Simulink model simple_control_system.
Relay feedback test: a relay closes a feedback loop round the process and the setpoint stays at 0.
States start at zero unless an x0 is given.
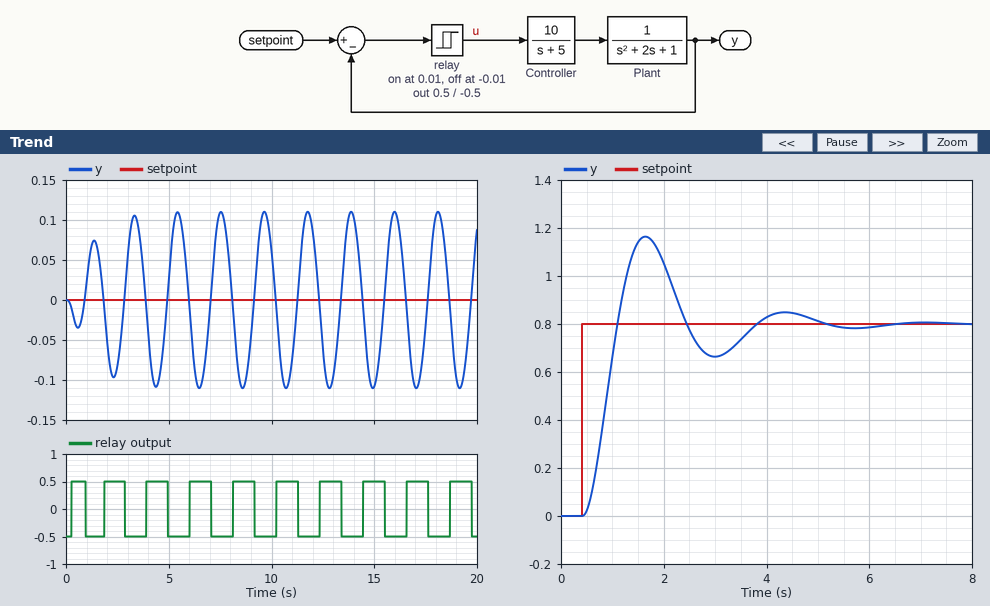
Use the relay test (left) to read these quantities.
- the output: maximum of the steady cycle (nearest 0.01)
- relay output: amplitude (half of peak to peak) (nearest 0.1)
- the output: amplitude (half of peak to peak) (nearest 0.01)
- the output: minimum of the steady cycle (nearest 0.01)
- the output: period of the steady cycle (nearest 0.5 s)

0.11
0.5
0.11
-0.11
2.0 s
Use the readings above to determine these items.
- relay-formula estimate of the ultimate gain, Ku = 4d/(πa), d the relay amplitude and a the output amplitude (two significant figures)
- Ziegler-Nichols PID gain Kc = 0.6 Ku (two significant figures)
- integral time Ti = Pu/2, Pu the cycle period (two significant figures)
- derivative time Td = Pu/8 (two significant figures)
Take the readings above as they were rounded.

5.8
3.5
1.0 s
0.25 s
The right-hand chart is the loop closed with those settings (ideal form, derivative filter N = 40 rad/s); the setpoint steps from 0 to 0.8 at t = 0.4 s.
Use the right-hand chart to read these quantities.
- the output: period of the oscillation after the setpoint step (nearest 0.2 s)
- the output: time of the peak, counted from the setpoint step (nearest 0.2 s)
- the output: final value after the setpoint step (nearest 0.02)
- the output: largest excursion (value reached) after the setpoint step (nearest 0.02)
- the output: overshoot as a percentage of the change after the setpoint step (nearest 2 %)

2.8 s
1.2 s
0.80
1.16
46 %
